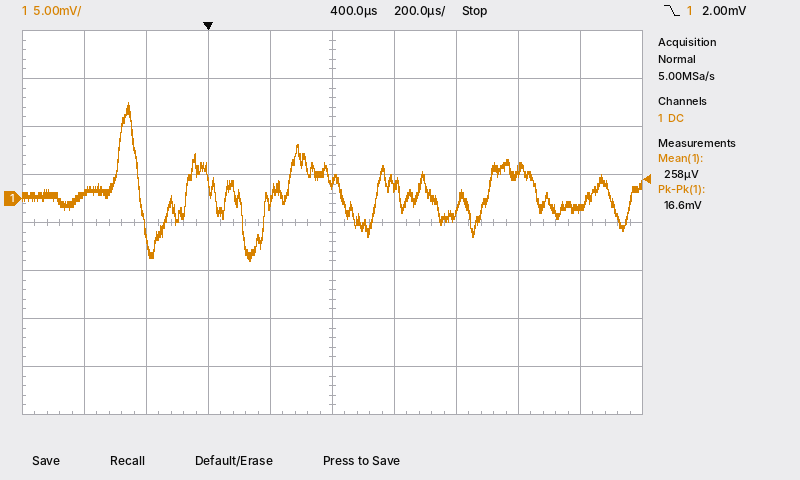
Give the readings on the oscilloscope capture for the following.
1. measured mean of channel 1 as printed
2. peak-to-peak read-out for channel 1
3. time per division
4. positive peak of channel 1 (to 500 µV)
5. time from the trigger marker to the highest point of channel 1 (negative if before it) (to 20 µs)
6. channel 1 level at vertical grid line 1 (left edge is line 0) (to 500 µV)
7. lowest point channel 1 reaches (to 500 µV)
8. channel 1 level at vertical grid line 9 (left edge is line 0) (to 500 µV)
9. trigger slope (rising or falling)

258 µV
16.6 mV
200 µs
10.0 mV
-260 µs
500 µV
-6.5 mV
-1.0 mV
falling
